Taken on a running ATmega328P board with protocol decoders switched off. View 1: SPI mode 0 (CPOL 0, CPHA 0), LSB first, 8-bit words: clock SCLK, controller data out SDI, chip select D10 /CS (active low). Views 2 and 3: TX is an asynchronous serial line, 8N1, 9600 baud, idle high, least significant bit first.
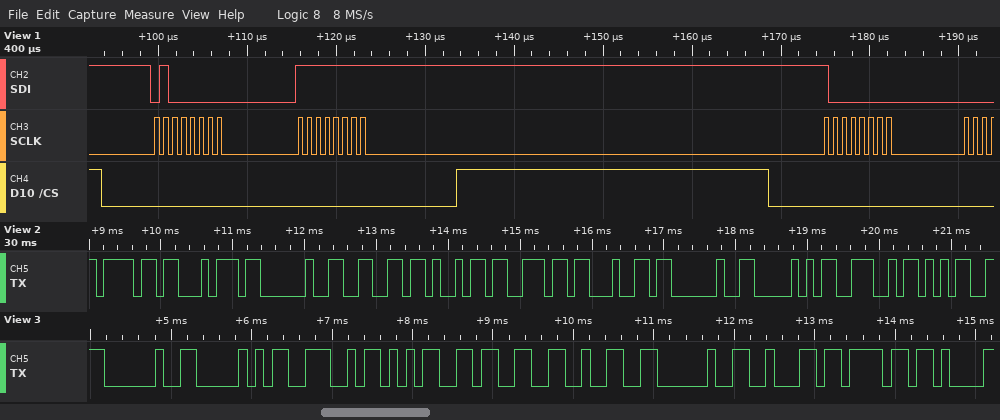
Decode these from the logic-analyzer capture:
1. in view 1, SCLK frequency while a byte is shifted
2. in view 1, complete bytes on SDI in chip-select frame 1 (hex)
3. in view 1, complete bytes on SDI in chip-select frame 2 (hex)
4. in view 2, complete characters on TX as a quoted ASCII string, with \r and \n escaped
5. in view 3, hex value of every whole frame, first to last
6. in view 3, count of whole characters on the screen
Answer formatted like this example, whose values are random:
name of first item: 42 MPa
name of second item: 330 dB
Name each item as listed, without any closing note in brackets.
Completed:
in view 1, SCLK frequency while a byte is shifted: 1 MHz
in view 1, complete bytes on SDI in chip-select frame 1: 02 FF
in view 1, complete bytes on SDI in chip-select frame 2: 01
in view 2, complete characters on TX as a quoted ASCII string, with \r and \n escaped: "ot find PN5"
in view 3, hex value of every whole frame, first to last: 0x20 0x50 0x4E 0x35 0x33 0x32 0x20 0x62 0x6F
in view 3, count of whole characters on the screen: 9
